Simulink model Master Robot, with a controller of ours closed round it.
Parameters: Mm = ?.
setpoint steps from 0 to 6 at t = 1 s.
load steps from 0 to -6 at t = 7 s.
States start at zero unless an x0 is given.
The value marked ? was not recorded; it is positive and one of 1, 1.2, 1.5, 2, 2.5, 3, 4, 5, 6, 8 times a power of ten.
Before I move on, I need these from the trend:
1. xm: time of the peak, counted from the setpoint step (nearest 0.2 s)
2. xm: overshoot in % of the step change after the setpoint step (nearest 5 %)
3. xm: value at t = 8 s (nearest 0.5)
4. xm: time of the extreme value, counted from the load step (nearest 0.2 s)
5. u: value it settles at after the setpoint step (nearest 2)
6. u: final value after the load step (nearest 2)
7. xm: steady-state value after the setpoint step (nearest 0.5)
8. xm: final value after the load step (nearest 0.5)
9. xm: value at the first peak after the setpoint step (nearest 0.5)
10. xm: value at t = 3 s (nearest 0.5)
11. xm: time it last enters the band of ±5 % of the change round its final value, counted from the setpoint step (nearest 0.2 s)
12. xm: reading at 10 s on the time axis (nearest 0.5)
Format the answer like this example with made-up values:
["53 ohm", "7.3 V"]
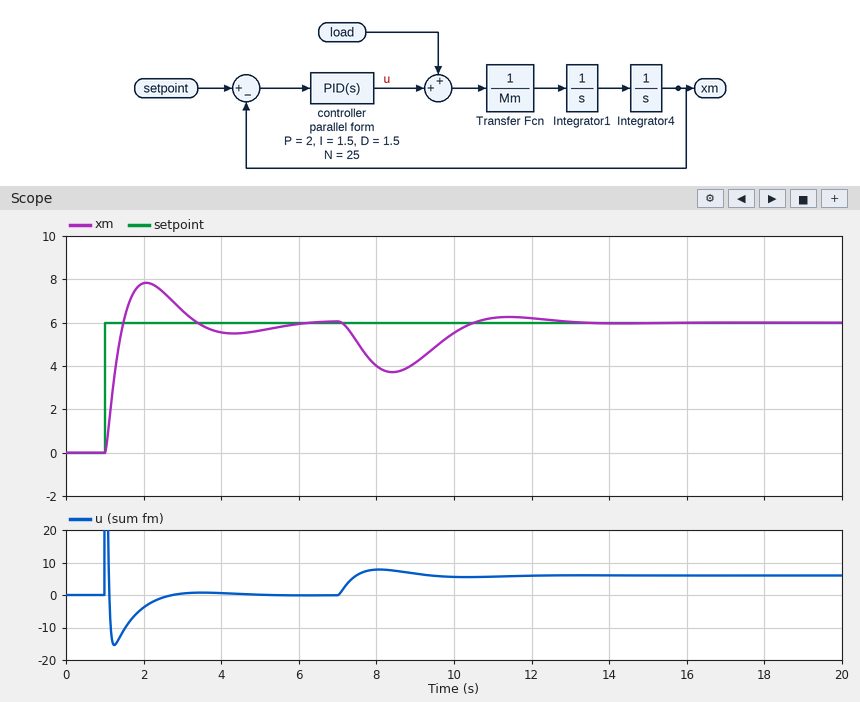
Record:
["1.0 s", "30 %", "4.0", "1.4 s", "0", "6", "6.0", "6.0", "8.0", "6.5", "4.2 s", "5.5"]
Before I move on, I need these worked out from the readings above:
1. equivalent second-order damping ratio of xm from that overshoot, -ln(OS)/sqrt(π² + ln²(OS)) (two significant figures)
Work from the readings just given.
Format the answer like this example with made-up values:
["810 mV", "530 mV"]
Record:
["0.36"]
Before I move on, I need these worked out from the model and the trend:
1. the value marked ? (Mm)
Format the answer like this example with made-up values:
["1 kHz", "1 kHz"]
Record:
["0.5"]
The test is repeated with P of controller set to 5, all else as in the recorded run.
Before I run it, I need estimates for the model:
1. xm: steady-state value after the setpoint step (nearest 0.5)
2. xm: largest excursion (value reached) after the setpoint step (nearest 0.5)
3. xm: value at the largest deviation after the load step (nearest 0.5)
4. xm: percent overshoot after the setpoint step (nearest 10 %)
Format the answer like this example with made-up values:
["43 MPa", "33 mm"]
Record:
["6.0", "8.5", "4.5", "40 %"]
